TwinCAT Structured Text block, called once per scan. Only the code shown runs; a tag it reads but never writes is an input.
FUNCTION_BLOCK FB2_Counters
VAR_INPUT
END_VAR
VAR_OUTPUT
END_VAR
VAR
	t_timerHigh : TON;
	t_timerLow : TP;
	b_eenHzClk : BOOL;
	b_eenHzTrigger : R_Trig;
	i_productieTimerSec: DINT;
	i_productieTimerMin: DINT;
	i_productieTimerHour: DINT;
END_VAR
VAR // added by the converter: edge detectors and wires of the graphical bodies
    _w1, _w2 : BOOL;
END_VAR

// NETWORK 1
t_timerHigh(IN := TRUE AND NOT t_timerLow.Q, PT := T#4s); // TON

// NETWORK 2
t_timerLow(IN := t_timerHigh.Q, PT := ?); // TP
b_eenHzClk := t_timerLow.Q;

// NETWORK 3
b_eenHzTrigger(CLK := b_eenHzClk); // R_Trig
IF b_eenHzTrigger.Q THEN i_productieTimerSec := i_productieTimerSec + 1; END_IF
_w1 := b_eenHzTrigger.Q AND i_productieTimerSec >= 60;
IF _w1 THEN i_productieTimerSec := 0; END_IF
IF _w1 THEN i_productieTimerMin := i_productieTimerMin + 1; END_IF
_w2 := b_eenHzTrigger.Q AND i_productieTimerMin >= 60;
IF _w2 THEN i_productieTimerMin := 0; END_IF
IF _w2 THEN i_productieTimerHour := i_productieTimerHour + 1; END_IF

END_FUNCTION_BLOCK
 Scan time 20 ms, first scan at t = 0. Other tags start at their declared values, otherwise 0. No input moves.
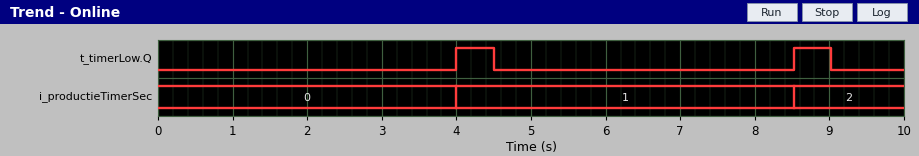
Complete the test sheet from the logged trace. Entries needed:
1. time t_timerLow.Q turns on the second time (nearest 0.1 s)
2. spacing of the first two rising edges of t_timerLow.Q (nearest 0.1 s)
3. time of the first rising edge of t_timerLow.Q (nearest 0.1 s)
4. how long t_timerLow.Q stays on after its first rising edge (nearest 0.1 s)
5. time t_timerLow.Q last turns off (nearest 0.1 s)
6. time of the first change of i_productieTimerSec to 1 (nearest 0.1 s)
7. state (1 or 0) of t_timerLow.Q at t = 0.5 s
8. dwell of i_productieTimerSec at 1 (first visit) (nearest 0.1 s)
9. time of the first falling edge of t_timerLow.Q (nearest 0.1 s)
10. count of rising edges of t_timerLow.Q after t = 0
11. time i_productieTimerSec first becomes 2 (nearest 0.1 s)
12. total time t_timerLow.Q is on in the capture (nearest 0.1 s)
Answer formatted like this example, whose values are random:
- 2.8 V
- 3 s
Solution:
- 8.5 s
- 4.5 s
- 4.0 s
- 0.5 s
- 9.0 s
- 4.0 s
- 0
- 4.5 s
- 4.5 s
- 2
- 8.5 s
- 1.0 s
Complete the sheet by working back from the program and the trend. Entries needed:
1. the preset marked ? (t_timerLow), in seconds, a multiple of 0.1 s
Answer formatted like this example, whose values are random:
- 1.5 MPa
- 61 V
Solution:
- 0.5 s
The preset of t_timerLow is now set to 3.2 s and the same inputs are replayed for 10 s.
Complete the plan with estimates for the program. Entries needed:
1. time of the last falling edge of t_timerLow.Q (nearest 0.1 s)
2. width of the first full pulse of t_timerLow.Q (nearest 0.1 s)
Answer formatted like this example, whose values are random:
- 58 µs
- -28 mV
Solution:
- 7.2 s
- 3.2 s
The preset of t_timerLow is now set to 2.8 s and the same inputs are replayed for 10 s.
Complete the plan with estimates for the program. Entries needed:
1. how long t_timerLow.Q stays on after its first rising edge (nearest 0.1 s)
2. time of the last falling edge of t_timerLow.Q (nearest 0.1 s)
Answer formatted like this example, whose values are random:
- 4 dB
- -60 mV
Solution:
- 2.8 s
- 6.8 s
